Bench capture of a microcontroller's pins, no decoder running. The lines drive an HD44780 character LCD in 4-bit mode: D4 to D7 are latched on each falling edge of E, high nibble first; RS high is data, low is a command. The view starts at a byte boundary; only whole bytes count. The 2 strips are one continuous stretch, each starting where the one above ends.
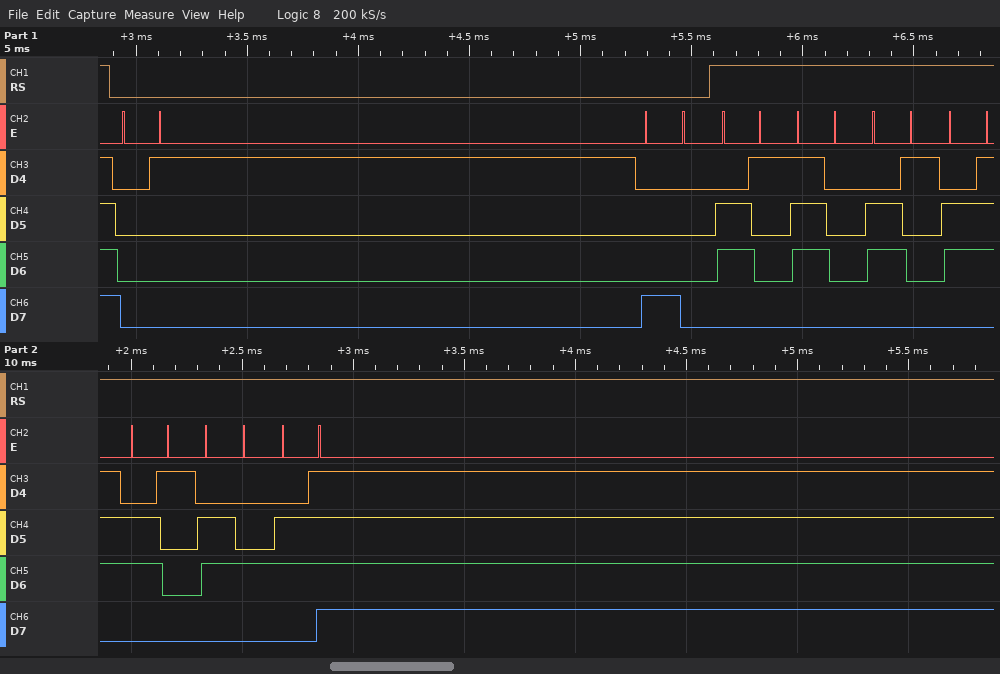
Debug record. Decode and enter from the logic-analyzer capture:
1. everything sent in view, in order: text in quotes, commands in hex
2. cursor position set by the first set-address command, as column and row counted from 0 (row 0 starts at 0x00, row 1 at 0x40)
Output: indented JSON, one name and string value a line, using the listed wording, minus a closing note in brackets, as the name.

{
  "everything sent in view, in order: text in quotes, commands in hex": "0x01 0x80 \"apagado\"",
  "cursor position set by the first set-address command, as column and row counted from 0": "column 0, row 0"
}
